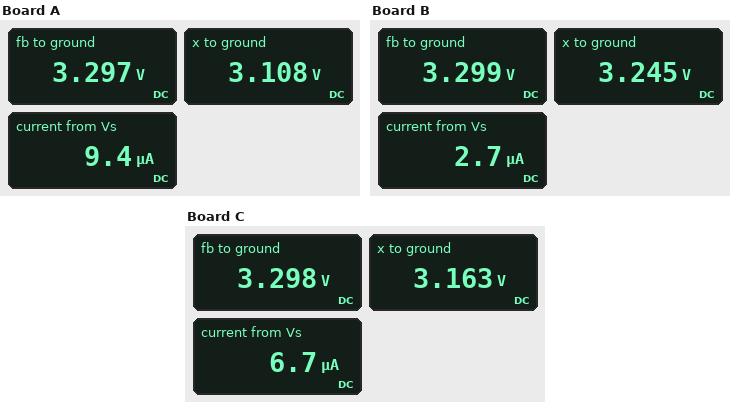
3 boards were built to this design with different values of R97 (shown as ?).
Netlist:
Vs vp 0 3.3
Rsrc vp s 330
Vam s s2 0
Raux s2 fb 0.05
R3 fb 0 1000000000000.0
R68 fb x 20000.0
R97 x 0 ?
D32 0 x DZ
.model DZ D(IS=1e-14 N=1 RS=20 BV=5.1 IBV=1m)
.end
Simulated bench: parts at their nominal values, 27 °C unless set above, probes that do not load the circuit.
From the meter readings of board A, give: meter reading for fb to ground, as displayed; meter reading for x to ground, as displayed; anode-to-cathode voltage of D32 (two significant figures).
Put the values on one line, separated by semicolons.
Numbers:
3.297 V; 3.108 V; -3.1 V
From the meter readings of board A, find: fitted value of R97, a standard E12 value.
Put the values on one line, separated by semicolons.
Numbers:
330 kΩ
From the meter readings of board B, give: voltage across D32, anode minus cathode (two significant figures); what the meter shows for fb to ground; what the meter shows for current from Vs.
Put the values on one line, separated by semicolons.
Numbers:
-3.2 V; 3.299 V; 2.7 µA
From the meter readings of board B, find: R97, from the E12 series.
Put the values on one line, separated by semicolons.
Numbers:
1.2 MΩ
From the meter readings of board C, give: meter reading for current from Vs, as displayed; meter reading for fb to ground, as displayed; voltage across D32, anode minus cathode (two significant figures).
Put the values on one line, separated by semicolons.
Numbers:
6.7 µA; 3.298 V; -3.2 V
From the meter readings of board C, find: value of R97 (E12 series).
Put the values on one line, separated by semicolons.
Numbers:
470 kΩ
